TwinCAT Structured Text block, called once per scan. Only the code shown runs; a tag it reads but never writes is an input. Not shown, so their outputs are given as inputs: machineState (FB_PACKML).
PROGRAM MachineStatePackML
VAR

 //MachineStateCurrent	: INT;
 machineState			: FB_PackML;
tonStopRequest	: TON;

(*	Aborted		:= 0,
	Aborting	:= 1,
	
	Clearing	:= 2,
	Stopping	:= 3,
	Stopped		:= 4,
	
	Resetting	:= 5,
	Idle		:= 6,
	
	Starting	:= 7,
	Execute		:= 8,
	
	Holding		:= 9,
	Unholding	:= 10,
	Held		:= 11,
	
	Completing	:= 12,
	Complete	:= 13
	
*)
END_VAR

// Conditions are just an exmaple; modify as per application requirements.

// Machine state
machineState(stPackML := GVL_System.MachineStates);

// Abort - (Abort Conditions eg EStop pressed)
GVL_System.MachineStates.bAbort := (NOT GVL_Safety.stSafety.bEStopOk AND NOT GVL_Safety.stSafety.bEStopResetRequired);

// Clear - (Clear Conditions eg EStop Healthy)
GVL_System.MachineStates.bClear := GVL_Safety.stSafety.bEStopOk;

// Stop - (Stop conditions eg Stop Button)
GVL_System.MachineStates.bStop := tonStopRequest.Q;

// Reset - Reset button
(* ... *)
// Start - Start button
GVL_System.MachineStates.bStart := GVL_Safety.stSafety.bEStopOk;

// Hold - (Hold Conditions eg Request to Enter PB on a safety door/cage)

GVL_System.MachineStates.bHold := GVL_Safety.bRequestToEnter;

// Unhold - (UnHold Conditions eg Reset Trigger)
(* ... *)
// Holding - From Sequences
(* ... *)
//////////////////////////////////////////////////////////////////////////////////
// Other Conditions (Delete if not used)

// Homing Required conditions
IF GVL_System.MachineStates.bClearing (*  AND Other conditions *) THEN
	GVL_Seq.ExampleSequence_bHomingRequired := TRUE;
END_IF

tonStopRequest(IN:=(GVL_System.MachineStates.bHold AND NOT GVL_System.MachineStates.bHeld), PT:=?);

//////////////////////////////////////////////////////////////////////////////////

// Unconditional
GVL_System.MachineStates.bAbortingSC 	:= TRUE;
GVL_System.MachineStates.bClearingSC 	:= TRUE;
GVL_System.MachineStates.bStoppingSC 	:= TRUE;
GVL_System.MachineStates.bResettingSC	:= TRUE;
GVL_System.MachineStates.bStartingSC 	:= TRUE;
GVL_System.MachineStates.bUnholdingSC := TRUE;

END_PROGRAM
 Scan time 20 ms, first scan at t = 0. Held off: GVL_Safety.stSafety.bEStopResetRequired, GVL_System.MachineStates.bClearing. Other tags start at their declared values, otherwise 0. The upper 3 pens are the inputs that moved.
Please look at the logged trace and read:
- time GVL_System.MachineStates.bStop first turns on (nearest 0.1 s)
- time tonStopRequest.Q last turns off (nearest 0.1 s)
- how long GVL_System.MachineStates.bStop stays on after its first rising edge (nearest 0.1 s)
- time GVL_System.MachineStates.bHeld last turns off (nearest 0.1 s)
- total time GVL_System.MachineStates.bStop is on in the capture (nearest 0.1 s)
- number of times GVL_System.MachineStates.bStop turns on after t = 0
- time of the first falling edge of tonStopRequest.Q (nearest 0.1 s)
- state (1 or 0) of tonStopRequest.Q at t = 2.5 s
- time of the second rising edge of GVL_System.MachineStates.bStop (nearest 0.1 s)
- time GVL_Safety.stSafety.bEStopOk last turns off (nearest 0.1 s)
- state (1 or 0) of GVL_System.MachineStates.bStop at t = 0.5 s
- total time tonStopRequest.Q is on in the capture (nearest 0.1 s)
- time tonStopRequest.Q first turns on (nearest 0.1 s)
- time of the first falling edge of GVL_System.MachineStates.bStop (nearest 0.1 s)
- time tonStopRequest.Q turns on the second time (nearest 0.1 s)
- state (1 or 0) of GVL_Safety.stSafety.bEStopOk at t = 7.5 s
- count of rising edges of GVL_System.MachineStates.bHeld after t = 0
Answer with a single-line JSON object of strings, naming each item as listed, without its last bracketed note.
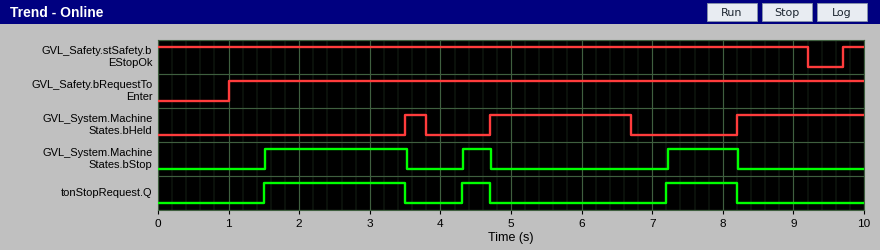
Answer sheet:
{"time GVL_System.MachineStates.bStop first turns on": "1.5 s", "time tonStopRequest.Q last turns off": "8.2 s", "how long GVL_System.MachineStates.bStop stays on after its first rising edge": "2.0 s", "time GVL_System.MachineStates.bHeld last turns off": "6.7 s", "total time GVL_System.MachineStates.bStop is on in the capture": "3.4 s", "number of times GVL_System.MachineStates.bStop turns on after t = 0": "3", "time of the first falling edge of tonStopRequest.Q": "3.5 s", "state (1 or 0) of tonStopRequest.Q at t = 2.5 s": "1", "time of the second rising edge of GVL_System.MachineStates.bStop": "4.3 s", "time GVL_Safety.stSafety.bEStopOk last turns off": "9.2 s", "state (1 or 0) of GVL_System.MachineStates.bStop at t = 0.5 s": "0", "total time tonStopRequest.Q is on in the capture": "3.4 s", "time tonStopRequest.Q first turns on": "1.5 s", "time of the first falling edge of GVL_System.MachineStates.bStop": "3.5 s", "time tonStopRequest.Q turns on the second time": "4.3 s", "state (1 or 0) of GVL_Safety.stSafety.bEStopOk at t = 7.5 s": "1", "count of rising edges of GVL_System.MachineStates.bHeld after t = 0": "3"}
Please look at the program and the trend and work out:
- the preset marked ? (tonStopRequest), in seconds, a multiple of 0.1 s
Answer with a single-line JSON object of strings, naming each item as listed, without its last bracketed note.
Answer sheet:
{"the preset marked ? (tonStopRequest), in seconds, a multiple of 0.1 s": "0.5 s"}
